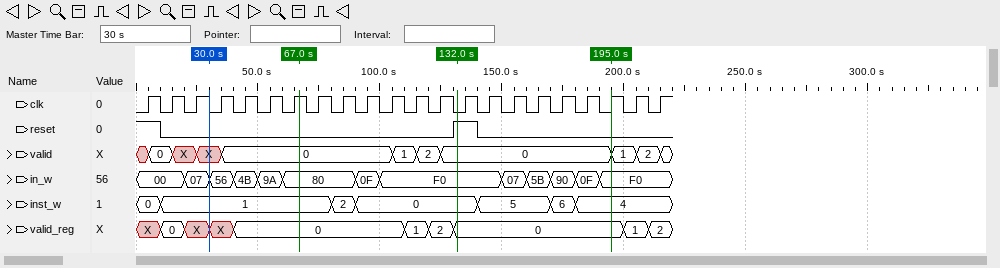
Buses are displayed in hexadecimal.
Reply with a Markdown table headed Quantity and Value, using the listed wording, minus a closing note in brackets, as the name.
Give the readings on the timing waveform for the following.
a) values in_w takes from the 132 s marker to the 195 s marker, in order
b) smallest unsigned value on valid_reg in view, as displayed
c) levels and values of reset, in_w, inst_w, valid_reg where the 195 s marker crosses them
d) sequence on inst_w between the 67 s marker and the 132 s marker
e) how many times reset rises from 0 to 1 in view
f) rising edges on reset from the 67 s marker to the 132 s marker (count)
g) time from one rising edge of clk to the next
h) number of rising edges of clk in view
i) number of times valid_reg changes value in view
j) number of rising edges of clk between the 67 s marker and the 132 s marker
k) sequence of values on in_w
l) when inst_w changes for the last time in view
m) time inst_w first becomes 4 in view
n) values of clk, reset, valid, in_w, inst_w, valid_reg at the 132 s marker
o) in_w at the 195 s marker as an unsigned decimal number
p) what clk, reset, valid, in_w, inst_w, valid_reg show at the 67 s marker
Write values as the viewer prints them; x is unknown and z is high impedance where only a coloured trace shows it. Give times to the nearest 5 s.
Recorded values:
| Quantity | Value |
|---|---|
| values in_w takes from the 132 s marker to the 195 s marker, in order | F0, 07, 5B, 90, 0F, F0 |
| smallest unsigned value on valid_reg in view, as displayed | 0 |
| levels and values of reset, in_w, inst_w, valid_reg where the 195 s marker crosses them | reset=0, in_w=F0, inst_w=4, valid_reg=0 |
| sequence on inst_w between the 67 s marker and the 132 s marker | 1, 2, 0 |
| how many times reset rises from 0 to 1 in view | 1 |
| rising edges on reset from the 67 s marker to the 132 s marker | 1 |
| time from one rising edge of clk to the next | 10 s |
| number of rising edges of clk in view | 22 |
| number of times valid_reg changes value in view | 9 |
| number of rising edges of clk between the 67 s marker and the 132 s marker | 6 |
| sequence of values on in_w | 00, 07, 56, 4B, 9A, 80, 0F, F0, 07, 5B, 90, 0F, F0 |
| when inst_w changes for the last time in view | 180 s |
| time inst_w first becomes 4 in view | 180 s |
| values of clk, reset, valid, in_w, inst_w, valid_reg at the 132 s marker | clk=0, reset=1, valid=0, in_w=F0, inst_w=0, valid_reg=0 |
| in_w at the 195 s marker as an unsigned decimal number | 240 |
| what clk, reset, valid, in_w, inst_w, valid_reg show at the 67 s marker | clk=1, reset=0, valid=0, in_w=80, inst_w=1, valid_reg=0 |
